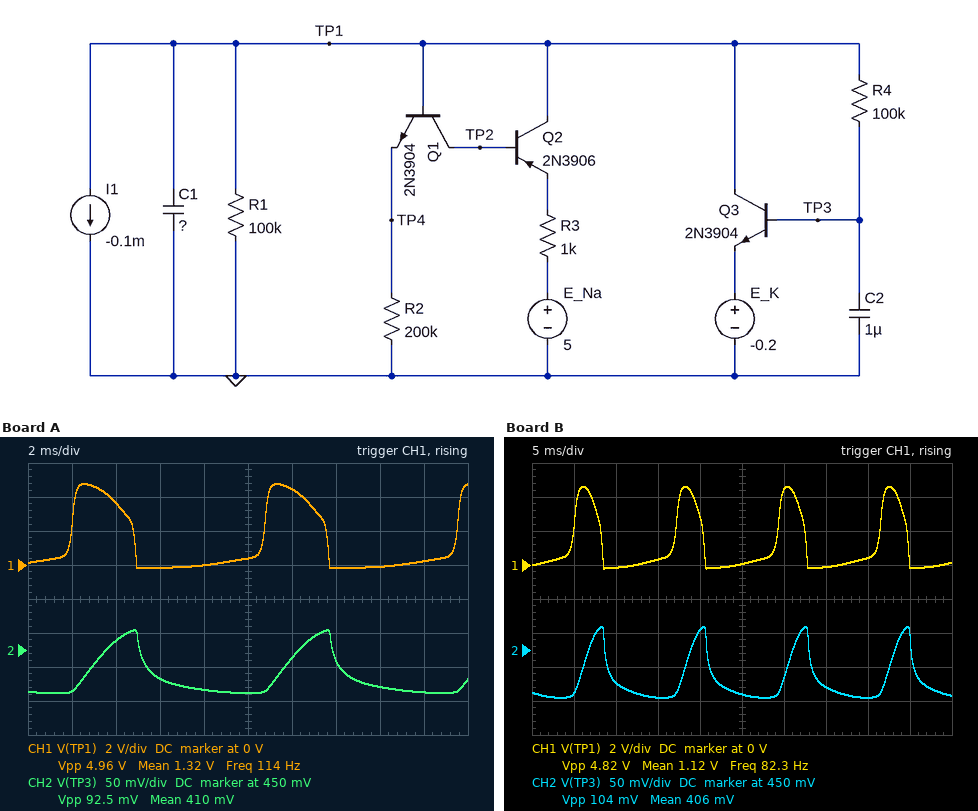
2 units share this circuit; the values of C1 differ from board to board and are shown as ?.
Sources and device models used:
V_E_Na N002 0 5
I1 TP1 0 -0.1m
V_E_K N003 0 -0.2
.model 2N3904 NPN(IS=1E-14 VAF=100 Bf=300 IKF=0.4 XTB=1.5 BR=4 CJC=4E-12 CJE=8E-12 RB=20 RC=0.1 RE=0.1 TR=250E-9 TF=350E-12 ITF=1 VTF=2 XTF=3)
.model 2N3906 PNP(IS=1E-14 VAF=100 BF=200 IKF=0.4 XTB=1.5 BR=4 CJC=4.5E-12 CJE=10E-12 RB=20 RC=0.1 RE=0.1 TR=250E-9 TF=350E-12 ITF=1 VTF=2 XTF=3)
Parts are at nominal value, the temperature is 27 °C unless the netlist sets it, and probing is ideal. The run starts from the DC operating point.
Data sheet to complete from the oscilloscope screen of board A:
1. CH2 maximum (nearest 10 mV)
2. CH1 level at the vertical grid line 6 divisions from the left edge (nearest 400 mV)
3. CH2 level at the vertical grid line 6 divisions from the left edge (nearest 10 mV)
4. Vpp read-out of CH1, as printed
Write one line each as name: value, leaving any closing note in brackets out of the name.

CH2 maximum: 480 mV
CH1 level at the vertical grid line 6 divisions from the left edge: 4.4 V
CH2 level at the vertical grid line 6 divisions from the left edge: 440 mV
Vpp read-out of CH1, as printed: 4.96 V
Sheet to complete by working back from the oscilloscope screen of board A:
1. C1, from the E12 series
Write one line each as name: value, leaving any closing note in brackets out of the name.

C1, from the E12 series: 120 nF
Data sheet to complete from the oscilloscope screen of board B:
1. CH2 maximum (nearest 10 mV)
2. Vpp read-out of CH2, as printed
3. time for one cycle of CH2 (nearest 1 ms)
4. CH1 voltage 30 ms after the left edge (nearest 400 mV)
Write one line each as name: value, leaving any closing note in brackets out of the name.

CH2 maximum: 480 mV
Vpp read-out of CH2, as printed: 104 mV
time for one cycle of CH2: 12 ms
CH1 voltage 30 ms after the left edge: 4.4 V
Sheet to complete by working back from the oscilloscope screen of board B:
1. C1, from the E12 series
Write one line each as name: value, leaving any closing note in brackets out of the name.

C1, from the E12 series: 330 nF
